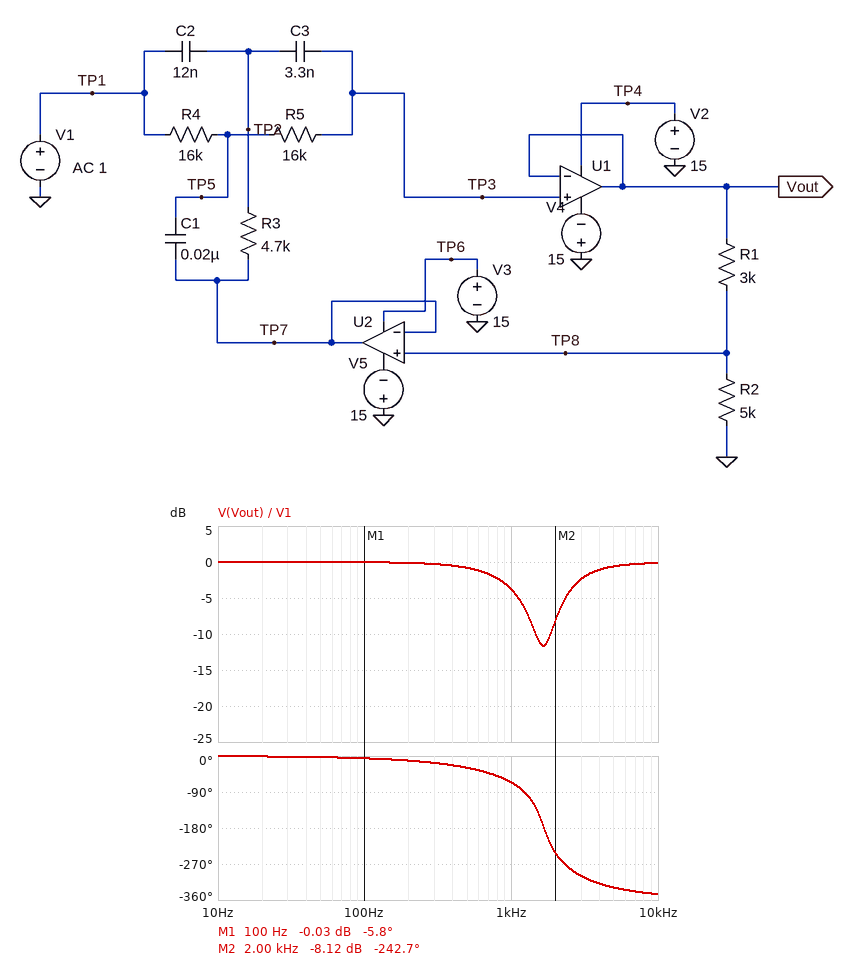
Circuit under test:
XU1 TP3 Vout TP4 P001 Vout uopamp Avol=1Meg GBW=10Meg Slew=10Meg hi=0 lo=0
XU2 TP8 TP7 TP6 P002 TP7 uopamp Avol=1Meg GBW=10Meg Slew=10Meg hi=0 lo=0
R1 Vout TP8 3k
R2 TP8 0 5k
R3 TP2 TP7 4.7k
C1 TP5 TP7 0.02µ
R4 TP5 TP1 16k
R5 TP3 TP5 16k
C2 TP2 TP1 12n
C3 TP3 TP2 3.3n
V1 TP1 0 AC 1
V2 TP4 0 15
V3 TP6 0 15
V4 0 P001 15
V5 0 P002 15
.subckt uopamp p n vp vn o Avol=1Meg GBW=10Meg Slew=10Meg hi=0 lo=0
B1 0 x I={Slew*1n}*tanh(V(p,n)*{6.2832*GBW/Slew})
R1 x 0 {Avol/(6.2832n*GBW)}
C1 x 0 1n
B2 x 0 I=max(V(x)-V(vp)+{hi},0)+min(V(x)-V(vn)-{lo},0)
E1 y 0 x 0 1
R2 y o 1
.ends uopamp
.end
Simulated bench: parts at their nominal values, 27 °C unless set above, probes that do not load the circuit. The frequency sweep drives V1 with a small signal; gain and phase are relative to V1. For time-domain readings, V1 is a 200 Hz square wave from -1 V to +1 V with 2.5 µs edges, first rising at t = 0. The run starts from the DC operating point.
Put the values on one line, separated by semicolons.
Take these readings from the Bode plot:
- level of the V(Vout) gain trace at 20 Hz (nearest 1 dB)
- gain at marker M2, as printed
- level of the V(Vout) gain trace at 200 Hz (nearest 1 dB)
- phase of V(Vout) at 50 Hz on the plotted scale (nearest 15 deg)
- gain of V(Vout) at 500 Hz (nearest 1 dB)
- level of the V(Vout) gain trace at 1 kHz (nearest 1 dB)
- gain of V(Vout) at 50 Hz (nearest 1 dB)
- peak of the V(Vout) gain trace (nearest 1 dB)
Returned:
0 dB; -8.12 dB; 0 dB; 0 deg; -1 dB; -4 dB; 0 dB; 0 dB
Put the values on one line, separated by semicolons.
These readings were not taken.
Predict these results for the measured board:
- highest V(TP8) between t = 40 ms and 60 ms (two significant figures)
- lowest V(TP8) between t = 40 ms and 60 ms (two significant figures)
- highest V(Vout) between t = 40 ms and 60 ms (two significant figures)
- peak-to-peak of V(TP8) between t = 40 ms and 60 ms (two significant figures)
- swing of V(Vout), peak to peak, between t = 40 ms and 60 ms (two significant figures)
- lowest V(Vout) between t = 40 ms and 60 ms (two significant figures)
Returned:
680 mV; -680 mV; 1.1 V; 1.4 V; 2.2 V; -1.1 V
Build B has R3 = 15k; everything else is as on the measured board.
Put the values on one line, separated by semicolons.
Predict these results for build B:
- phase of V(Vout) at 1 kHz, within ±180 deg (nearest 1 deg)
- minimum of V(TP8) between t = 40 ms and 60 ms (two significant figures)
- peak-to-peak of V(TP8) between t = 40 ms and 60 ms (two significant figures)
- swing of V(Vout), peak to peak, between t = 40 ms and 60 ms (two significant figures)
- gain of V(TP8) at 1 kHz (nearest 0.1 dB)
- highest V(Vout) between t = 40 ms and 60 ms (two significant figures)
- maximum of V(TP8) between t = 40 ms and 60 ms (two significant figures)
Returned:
-53 deg; -650 mV; 1.3 V; 2.1 V; -12.9 dB; 1.0 V; 650 mV
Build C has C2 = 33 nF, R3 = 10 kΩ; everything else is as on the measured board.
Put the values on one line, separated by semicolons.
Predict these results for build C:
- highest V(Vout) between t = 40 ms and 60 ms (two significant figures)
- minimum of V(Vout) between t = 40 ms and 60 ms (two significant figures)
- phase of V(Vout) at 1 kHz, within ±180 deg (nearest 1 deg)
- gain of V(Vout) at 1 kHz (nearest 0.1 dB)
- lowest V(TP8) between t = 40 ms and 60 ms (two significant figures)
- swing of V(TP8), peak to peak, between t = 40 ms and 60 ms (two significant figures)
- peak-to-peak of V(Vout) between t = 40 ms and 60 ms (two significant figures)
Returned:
1.0 V; -1.0 V; -28 deg; -9.8 dB; -640 mV; 1.3 V; 2.0 V
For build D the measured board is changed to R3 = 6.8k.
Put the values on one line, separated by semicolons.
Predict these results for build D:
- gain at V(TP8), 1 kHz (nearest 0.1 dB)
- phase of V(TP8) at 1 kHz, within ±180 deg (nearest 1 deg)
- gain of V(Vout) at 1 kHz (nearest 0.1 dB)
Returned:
-9.2 dB; -68 deg; -5.1 dB
